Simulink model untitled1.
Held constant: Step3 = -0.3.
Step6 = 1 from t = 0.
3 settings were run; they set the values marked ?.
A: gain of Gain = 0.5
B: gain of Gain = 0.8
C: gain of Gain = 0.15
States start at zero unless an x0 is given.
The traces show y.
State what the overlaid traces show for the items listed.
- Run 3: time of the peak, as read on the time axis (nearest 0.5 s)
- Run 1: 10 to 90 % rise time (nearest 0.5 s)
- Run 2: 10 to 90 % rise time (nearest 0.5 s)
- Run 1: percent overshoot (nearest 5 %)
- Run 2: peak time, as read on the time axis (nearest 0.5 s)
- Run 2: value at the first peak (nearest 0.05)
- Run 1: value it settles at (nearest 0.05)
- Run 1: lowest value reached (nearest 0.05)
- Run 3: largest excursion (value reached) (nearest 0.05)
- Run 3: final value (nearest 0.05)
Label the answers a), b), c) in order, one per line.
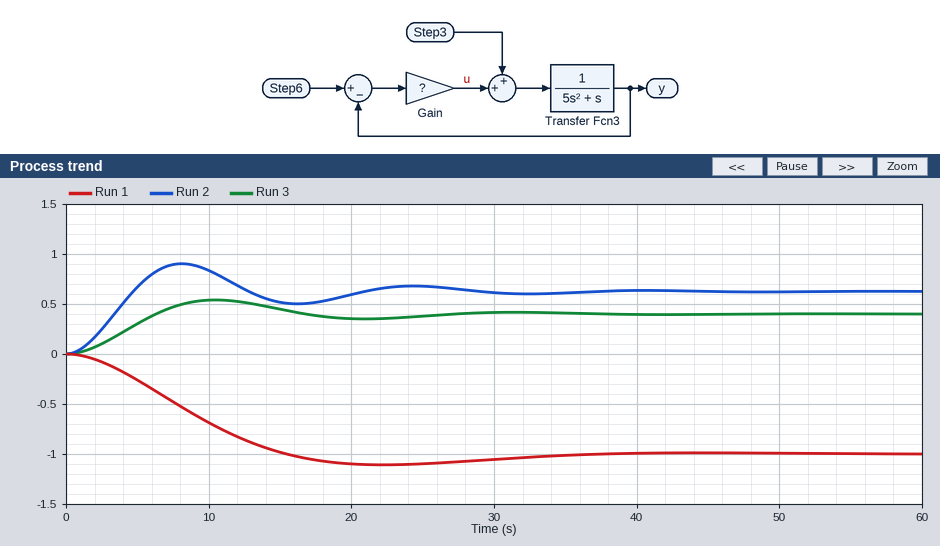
a) 10.5 s
b) 10.5 s
c) 3.0 s
d) 10 %
e) 8.0 s
f) 0.90
g) -1.00
h) -1.10
i) 0.55
j) 0.40
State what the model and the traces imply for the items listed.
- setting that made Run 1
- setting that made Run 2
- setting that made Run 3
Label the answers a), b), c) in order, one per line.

a) C
b) B
c) A
